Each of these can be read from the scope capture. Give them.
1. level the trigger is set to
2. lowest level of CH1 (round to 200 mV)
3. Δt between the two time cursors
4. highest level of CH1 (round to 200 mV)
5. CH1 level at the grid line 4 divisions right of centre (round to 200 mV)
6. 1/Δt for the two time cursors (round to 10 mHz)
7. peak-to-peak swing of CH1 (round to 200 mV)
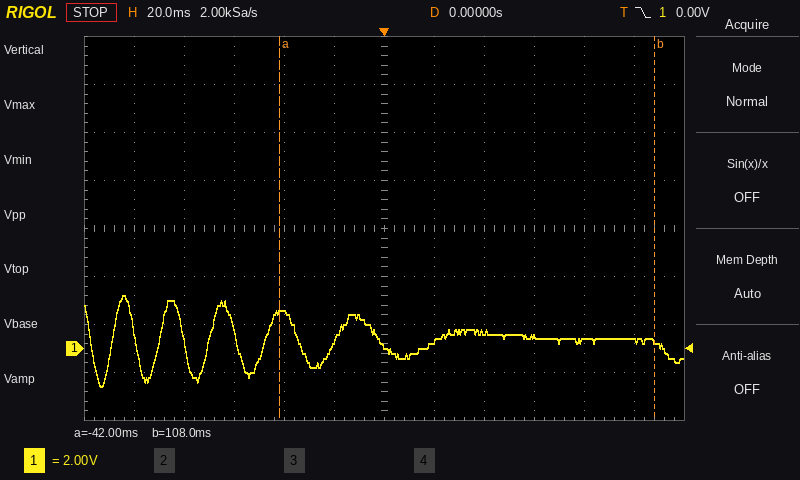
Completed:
0.00 V
-1.6 V
150 ms
2.2 V
400 mV
6.67 Hz
3.8 V
